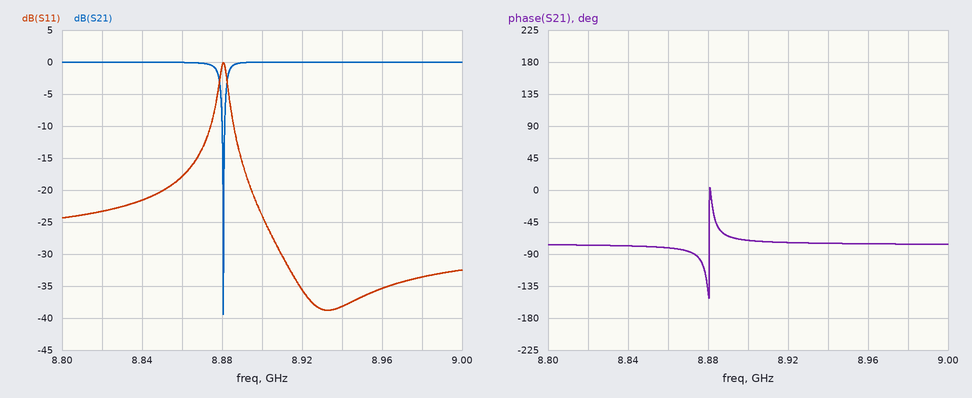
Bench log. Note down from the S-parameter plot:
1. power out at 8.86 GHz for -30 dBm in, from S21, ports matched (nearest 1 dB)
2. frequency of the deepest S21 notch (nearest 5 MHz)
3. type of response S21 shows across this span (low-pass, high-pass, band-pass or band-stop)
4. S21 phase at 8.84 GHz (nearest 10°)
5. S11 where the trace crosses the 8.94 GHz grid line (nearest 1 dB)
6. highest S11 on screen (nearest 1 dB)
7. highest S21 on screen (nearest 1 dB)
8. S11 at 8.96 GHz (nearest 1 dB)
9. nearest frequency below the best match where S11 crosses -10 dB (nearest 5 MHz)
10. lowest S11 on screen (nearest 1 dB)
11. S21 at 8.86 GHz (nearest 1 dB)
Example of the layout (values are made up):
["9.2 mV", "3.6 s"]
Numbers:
["-30 dBm", "8.880 GHz", "band-stop", "-80°", "-38 dB", "0 dB", "0 dB", "-35 dB", "8.885 GHz", "-39 dB", "0 dB"]
